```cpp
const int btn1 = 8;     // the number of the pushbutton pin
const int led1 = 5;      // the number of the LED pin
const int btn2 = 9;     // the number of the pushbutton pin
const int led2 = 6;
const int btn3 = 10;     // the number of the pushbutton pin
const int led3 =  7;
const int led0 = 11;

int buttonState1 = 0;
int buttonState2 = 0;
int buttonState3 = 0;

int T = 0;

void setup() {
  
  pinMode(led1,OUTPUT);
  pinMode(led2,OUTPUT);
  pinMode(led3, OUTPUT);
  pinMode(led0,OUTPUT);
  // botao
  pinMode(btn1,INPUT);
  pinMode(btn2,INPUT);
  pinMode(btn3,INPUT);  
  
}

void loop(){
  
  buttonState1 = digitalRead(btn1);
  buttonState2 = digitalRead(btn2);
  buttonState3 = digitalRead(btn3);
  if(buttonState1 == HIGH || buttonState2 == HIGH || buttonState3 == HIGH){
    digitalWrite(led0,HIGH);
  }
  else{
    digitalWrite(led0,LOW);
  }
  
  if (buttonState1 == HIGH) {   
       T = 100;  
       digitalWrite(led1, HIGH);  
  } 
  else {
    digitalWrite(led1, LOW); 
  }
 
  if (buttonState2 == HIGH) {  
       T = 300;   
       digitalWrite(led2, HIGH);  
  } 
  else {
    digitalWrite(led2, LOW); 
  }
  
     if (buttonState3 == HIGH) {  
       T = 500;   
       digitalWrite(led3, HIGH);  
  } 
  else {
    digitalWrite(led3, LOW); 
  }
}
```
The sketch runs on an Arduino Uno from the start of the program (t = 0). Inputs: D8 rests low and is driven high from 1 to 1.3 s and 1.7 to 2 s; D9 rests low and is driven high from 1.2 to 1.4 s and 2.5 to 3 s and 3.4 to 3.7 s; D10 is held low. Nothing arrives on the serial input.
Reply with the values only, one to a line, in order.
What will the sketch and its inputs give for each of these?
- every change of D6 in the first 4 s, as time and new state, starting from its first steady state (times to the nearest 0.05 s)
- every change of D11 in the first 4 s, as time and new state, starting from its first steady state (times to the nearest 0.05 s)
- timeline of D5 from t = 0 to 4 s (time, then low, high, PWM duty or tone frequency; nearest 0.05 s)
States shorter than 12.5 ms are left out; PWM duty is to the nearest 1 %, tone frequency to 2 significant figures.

0 s low; 1.2 s high; 1.4 s low; 2.5 s high; 3 s low; 3.4 s high; 3.7 s low
0 s low; 1 s high; 1.4 s low; 1.7 s high; 2 s low; 2.5 s high; 3 s low; 3.4 s high; 3.7 s low
0 s low; 1 s high; 1.3 s low; 1.7 s high; 2 s low
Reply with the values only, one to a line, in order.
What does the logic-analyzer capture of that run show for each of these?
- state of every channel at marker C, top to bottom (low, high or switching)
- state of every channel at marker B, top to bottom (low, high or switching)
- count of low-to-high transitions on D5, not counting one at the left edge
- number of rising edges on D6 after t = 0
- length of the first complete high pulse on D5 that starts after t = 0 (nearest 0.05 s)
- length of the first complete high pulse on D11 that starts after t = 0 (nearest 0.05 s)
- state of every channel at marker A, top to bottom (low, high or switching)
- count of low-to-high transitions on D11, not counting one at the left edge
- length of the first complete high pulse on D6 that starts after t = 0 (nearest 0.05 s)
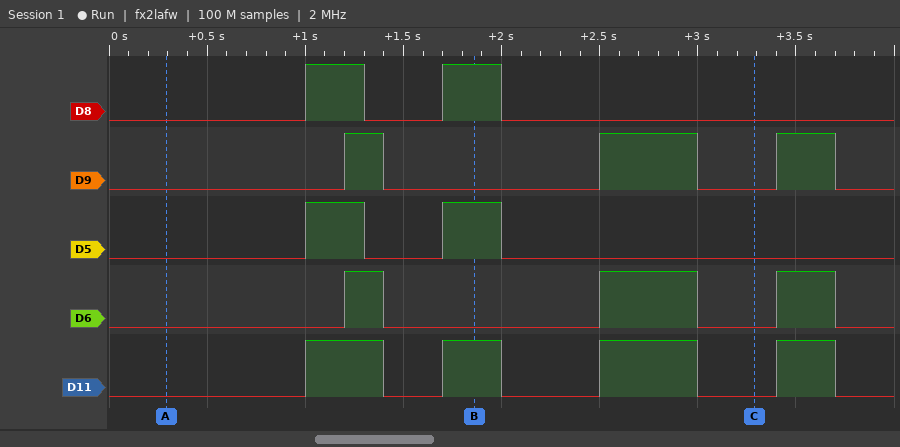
D8 low, D9 low, D5 low, D6 low, D11 low
D8 high, D9 low, D5 high, D6 low, D11 high
2
3
0.30 s
0.40 s
D8 low, D9 low, D5 low, D6 low, D11 low
4
0.20 s
